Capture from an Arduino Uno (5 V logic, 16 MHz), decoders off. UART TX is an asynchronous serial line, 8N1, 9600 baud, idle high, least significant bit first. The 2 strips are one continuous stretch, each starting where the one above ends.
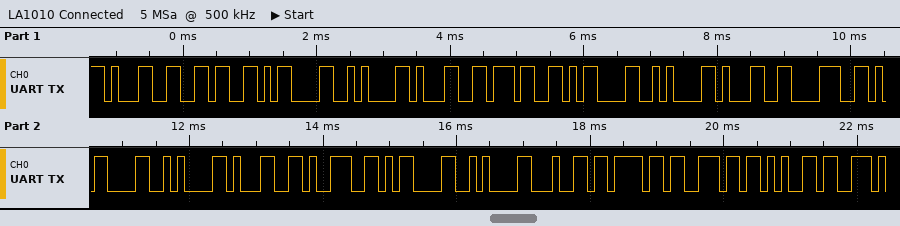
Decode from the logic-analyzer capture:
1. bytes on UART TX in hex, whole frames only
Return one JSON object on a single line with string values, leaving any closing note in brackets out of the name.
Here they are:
{"bytes on UART TX in hex, whole frames only": "31 36 0D 0A 31 37 0D 0A 31 38 0D 0A 31 39 0D 0A 64 6F 6E 65"}
